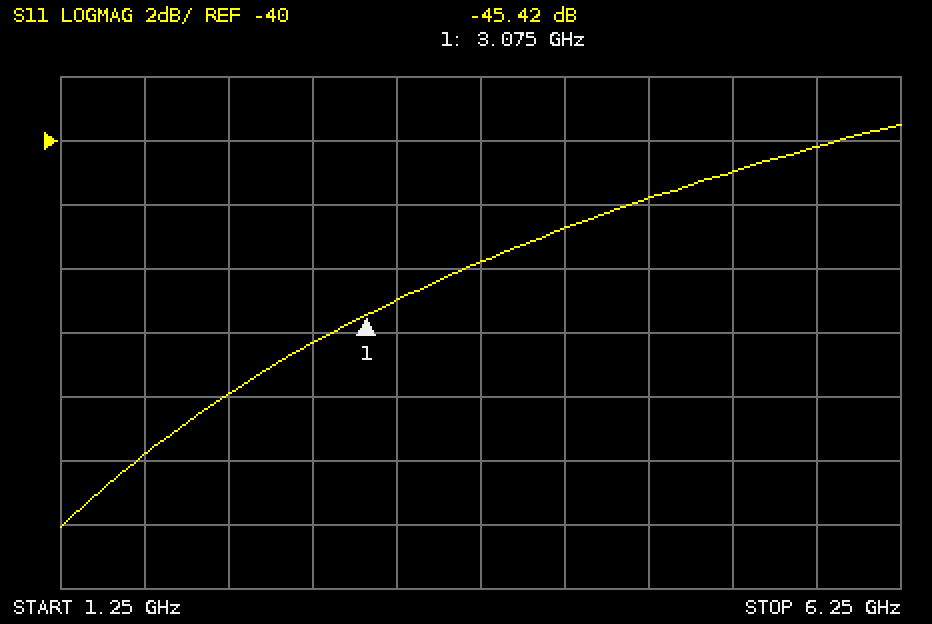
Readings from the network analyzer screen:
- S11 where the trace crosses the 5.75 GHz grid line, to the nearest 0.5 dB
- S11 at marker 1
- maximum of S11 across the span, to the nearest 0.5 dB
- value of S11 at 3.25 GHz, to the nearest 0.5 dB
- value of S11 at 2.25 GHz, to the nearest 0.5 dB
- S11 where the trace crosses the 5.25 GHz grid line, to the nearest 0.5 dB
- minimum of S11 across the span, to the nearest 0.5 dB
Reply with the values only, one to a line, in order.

-40.0 dB
-45.42 dB
-39.5 dB
-45.0 dB
-48.0 dB
-41.0 dB
-52.0 dB
